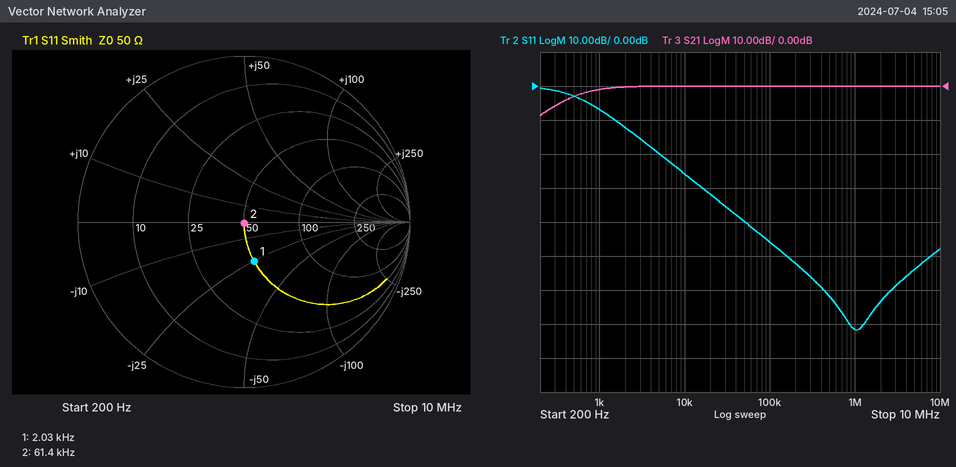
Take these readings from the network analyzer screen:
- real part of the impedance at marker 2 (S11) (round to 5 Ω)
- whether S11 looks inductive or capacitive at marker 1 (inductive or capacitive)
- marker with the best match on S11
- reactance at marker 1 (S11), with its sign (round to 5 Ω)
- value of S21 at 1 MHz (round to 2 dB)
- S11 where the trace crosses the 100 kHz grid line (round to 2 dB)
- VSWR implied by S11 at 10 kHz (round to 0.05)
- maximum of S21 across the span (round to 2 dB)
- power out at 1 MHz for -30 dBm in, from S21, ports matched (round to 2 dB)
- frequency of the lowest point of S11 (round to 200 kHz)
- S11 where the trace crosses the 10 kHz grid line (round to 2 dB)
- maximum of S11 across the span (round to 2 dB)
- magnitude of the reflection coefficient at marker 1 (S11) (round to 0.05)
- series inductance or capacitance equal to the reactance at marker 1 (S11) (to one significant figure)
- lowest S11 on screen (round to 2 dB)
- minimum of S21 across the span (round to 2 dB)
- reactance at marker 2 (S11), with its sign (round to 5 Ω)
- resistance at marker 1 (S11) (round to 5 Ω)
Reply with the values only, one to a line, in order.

50 Ω
capacitive
marker 2
-25 Ω
0 dB
-46 dB
1.10
0 dB
-30 dBm
1.0 MHz
-26 dB
0 dB
0.25
3 µF
-72 dB
-8 dB
0 Ω
50 Ω
